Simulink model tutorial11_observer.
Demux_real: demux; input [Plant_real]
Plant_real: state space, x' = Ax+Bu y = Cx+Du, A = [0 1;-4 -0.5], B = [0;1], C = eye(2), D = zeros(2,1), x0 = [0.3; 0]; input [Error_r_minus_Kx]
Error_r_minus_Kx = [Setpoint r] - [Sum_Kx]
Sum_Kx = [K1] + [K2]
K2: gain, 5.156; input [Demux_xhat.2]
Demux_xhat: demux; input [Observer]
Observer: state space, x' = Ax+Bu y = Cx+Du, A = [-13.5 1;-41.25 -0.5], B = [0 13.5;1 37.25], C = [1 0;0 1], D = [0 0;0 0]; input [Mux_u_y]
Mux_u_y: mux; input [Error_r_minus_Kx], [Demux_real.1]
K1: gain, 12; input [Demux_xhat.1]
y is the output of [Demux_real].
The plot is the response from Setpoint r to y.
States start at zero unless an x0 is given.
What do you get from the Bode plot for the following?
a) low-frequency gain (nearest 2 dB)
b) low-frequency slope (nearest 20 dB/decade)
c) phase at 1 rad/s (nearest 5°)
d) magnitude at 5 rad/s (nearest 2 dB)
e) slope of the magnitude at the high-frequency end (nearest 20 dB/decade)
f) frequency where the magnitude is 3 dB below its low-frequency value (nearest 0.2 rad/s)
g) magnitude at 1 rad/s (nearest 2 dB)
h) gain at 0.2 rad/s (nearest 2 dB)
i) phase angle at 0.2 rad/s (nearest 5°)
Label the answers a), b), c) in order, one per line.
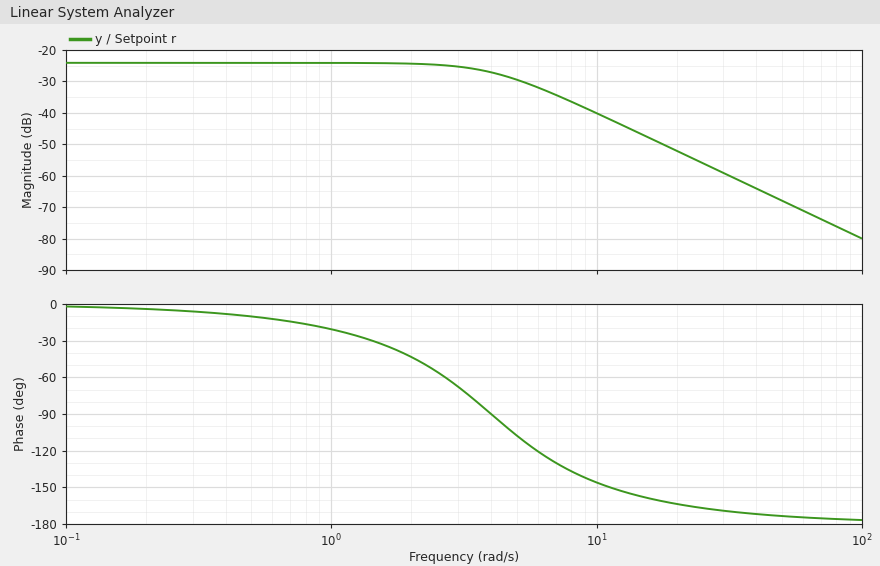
a) -24 dB
b) 0 dB/decade
c) -20°
d) -30 dB
e) -40 dB/decade
f) 4.0 rad/s
g) -24 dB
h) -24 dB
i) -5°
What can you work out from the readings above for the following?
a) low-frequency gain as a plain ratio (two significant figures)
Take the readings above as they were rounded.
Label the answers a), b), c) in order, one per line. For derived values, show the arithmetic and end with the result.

a) 10^(-24 / 20) = 0.063
